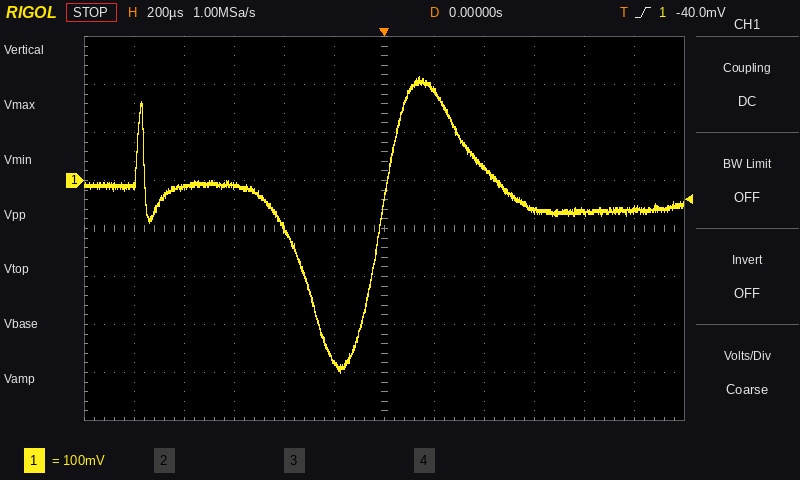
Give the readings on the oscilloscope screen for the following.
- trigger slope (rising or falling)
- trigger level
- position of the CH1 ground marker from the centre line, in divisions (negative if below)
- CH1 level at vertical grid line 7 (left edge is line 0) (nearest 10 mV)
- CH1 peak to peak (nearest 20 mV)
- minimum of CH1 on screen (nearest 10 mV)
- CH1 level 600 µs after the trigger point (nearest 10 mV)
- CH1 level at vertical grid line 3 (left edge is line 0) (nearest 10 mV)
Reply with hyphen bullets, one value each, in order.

- rising
- -40.0 mV
- +1.0 div
- 190 mV
- 620 mV
- -400 mV
- -60 mV
- -10 mV
